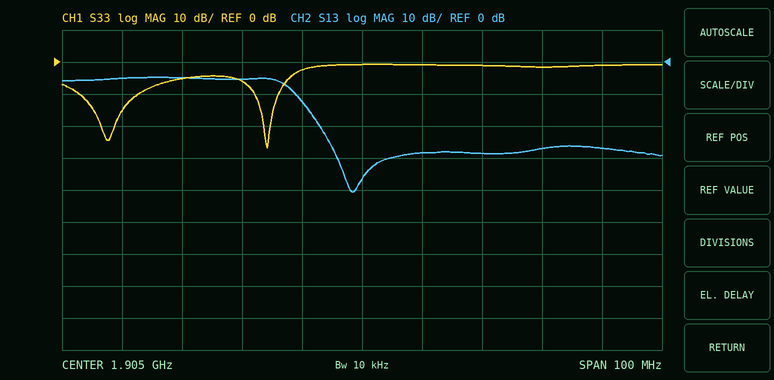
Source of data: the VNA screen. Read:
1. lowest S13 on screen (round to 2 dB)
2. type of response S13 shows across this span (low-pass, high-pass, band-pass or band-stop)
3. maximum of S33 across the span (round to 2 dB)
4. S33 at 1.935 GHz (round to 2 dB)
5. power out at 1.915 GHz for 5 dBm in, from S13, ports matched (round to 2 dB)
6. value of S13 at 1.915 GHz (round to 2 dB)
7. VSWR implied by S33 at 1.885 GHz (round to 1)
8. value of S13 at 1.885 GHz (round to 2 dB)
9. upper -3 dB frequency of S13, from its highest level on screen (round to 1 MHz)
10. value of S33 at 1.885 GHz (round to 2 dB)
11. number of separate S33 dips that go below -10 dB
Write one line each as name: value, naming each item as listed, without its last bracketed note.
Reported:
lowest S13 on screen: -40 dB
type of response S13 shows across this span: low-pass
maximum of S33 across the span: 0 dB
S33 at 1.935 GHz: -2 dB
power out at 1.915 GHz for 5 dBm in, from S13, ports matched: -24 dBm
value of S13 at 1.915 GHz: -28 dB
VSWR implied by S33 at 1.885 GHz: 3
value of S13 at 1.885 GHz: -6 dB
upper -3 dB frequency of S13, from its highest level on screen: 1.893 GHz
value of S33 at 1.885 GHz: -6 dB
number of separate S33 dips that go below -10 dB: 2
